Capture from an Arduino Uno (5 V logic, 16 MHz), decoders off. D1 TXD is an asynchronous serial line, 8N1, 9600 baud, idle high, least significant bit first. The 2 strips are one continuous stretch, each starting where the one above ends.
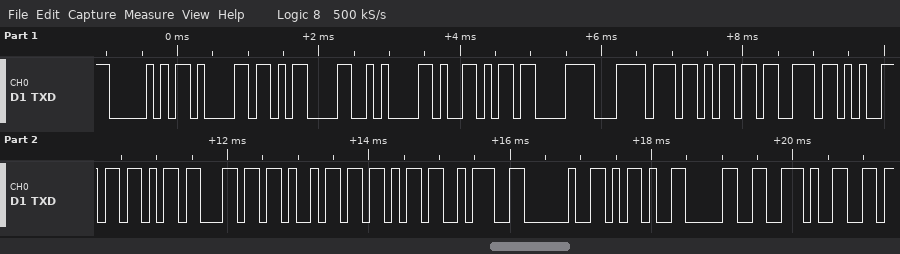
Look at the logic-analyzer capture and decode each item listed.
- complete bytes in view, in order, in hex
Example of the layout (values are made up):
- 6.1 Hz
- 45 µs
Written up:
- 0x50 0x61 0x0D 0x0A 0x59 0xC3 0xBC 0x6B 0x73 0x65 0x6B 0x6C 0x69 0x6B 0x3A 0x20 0x2D 0x30 0x2E
